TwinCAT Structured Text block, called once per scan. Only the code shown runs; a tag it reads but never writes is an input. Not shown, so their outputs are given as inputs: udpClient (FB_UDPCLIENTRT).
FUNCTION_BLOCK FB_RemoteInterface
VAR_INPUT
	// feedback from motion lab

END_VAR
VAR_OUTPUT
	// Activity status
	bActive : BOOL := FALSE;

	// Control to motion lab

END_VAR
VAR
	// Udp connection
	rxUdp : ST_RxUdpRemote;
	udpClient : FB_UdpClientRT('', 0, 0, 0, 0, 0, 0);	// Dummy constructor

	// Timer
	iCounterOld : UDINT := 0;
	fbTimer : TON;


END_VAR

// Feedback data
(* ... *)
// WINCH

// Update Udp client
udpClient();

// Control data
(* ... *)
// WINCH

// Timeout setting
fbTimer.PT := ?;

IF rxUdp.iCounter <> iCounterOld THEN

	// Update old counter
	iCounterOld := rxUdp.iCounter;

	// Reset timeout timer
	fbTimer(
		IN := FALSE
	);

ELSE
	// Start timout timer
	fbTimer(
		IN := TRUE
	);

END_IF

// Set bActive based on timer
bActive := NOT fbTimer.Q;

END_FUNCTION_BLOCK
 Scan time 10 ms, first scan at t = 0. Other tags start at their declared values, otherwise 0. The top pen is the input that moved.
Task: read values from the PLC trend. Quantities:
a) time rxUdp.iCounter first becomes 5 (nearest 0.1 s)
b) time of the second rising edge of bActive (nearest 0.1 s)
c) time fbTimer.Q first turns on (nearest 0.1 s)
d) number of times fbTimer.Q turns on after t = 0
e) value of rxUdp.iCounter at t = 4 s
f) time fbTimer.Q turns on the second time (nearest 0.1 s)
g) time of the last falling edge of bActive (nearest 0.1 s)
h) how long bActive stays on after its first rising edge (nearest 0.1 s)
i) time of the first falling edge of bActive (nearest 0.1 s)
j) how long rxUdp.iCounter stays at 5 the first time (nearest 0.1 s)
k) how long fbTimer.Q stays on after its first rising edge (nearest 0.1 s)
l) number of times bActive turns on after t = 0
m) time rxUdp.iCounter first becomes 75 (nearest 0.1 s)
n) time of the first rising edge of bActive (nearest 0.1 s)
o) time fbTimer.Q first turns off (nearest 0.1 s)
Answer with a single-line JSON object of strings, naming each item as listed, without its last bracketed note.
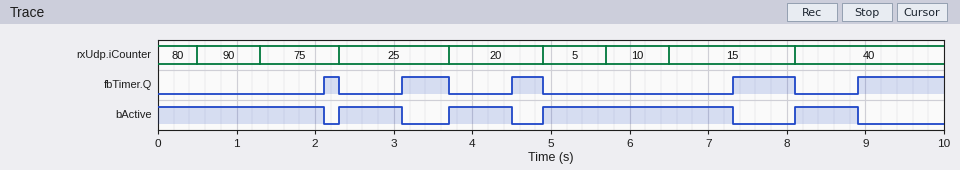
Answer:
{"time rxUdp.iCounter first becomes 5": "4.9 s", "time of the second rising edge of bActive": "3.7 s", "time fbTimer.Q first turns on": "2.1 s", "number of times fbTimer.Q turns on after t = 0": "5", "value of rxUdp.iCounter at t = 4 s": "20", "time fbTimer.Q turns on the second time": "3.1 s", "time of the last falling edge of bActive": "8.9 s", "how long bActive stays on after its first rising edge": "0.8 s", "time of the first falling edge of bActive": "2.1 s", "how long rxUdp.iCounter stays at 5 the first time": "0.8 s", "how long fbTimer.Q stays on after its first rising edge": "0.2 s", "number of times bActive turns on after t = 0": "4", "time rxUdp.iCounter first becomes 75": "1.3 s", "time of the first rising edge of bActive": "2.3 s", "time fbTimer.Q first turns off": "2.3 s"}
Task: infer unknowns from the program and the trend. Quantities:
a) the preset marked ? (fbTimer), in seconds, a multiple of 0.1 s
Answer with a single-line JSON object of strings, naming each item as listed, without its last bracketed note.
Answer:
{"the preset marked ? (fbTimer), in seconds, a multiple of 0.1 s": "0.8 s"}
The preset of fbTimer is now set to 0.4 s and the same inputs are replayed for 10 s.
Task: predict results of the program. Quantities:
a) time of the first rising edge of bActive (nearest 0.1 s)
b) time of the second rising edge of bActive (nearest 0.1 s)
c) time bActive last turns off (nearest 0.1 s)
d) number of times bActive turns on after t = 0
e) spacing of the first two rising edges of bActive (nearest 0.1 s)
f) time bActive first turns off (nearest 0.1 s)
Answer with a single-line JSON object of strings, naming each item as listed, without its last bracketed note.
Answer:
{"time of the first rising edge of bActive": "0.5 s", "time of the second rising edge of bActive": "1.3 s", "time bActive last turns off": "8.5 s", "number of times bActive turns on after t = 0": "8", "spacing of the first two rising edges of bActive": "0.8 s", "time bActive first turns off": "0.4 s"}
